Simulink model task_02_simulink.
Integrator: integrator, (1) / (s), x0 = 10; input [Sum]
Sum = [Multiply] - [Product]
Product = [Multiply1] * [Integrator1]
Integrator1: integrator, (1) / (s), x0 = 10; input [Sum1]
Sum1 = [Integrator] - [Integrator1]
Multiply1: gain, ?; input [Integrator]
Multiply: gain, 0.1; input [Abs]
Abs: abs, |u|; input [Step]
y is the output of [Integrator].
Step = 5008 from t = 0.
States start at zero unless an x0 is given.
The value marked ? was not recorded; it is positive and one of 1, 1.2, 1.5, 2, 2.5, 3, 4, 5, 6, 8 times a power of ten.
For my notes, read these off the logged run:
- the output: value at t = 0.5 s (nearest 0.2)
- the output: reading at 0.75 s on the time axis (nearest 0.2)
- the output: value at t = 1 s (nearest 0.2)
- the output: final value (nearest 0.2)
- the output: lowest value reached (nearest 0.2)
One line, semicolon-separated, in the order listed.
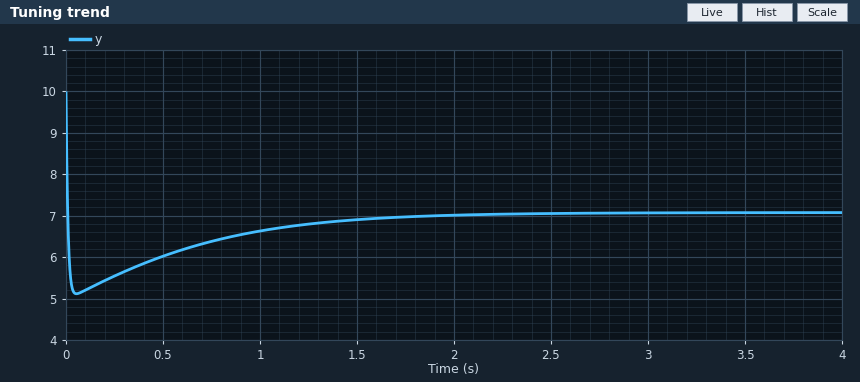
6.0; 6.4; 6.6; 7.0; 5.2
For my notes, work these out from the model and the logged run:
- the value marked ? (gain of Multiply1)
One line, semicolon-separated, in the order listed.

10
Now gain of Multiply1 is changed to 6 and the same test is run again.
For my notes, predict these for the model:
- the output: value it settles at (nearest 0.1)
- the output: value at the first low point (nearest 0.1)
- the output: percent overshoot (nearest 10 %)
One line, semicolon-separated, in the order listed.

9.1; 8.4; 80 %
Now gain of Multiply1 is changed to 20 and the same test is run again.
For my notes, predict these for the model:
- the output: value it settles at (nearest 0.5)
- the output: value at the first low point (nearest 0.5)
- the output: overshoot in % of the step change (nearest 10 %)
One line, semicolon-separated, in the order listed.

5.0; 2.5; 50 %
